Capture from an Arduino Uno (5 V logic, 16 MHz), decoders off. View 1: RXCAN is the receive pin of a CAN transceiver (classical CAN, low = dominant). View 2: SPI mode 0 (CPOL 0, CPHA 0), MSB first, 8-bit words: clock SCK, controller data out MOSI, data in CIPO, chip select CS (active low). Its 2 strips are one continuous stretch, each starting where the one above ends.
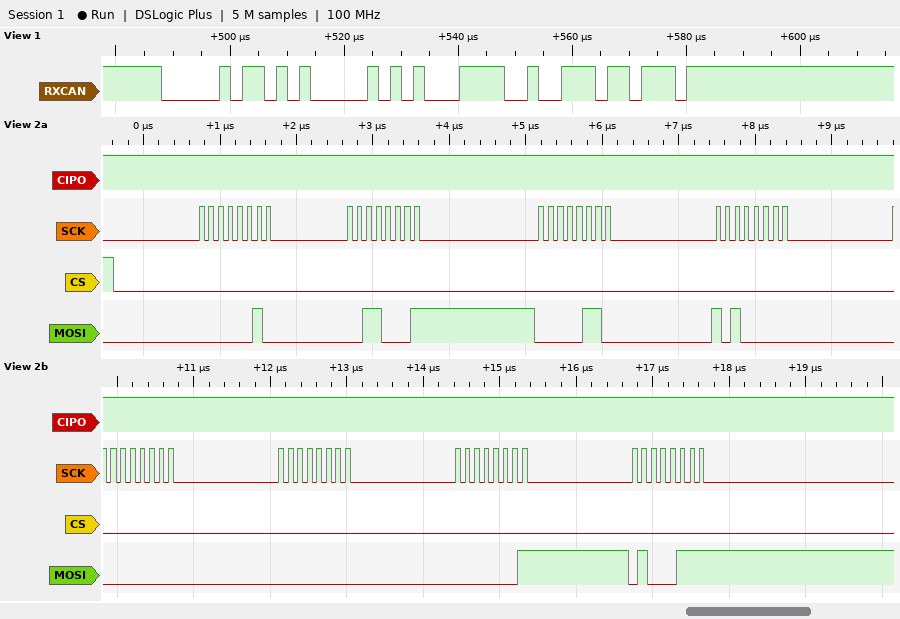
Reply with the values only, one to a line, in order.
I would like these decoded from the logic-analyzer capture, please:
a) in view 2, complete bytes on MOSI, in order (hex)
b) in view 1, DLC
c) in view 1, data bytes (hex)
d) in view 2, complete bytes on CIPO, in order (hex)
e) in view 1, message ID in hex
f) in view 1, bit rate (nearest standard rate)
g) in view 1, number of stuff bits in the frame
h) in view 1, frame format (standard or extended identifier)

0x02 0x31 0x06 0xA0 0x00 0x00 0x01 0x47
1
47
0xFF 0xFF 0xFF 0xFF 0xFF 0xFF 0xFF 0xFF
0x035
500 kbit/s
2
standard
